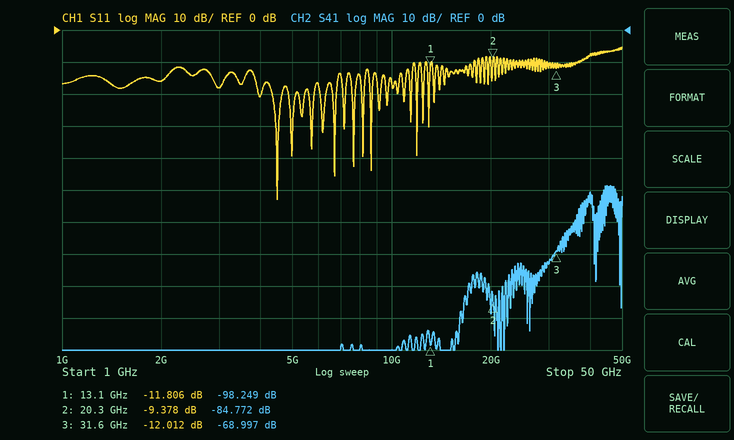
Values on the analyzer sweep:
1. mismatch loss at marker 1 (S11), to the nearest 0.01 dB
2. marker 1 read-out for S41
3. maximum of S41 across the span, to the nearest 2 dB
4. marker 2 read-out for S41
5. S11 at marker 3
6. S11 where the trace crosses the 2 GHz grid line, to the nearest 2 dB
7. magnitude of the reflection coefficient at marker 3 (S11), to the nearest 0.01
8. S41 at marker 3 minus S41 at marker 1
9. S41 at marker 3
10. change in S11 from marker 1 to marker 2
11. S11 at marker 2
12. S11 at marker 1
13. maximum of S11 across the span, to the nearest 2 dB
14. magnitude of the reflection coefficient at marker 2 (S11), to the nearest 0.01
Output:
0.30 dB
-98.249 dB
-48 dB
-84.772 dB
-12.012 dB
-16 dB
0.25
29.252 dB
-68.997 dB
2.428 dB
-9.378 dB
-11.806 dB
-6 dB
0.34
